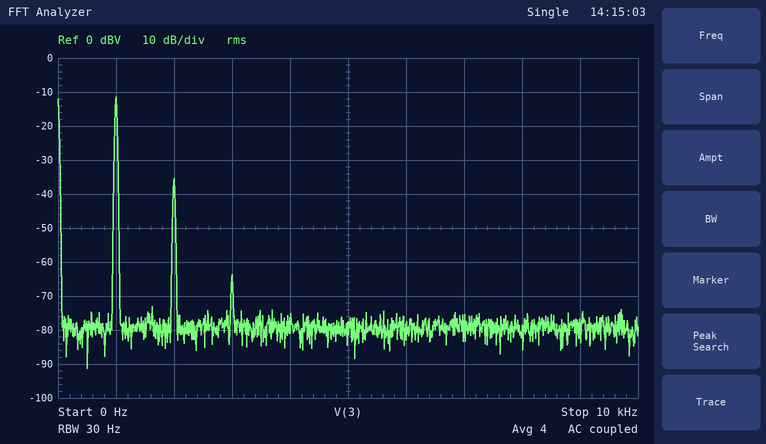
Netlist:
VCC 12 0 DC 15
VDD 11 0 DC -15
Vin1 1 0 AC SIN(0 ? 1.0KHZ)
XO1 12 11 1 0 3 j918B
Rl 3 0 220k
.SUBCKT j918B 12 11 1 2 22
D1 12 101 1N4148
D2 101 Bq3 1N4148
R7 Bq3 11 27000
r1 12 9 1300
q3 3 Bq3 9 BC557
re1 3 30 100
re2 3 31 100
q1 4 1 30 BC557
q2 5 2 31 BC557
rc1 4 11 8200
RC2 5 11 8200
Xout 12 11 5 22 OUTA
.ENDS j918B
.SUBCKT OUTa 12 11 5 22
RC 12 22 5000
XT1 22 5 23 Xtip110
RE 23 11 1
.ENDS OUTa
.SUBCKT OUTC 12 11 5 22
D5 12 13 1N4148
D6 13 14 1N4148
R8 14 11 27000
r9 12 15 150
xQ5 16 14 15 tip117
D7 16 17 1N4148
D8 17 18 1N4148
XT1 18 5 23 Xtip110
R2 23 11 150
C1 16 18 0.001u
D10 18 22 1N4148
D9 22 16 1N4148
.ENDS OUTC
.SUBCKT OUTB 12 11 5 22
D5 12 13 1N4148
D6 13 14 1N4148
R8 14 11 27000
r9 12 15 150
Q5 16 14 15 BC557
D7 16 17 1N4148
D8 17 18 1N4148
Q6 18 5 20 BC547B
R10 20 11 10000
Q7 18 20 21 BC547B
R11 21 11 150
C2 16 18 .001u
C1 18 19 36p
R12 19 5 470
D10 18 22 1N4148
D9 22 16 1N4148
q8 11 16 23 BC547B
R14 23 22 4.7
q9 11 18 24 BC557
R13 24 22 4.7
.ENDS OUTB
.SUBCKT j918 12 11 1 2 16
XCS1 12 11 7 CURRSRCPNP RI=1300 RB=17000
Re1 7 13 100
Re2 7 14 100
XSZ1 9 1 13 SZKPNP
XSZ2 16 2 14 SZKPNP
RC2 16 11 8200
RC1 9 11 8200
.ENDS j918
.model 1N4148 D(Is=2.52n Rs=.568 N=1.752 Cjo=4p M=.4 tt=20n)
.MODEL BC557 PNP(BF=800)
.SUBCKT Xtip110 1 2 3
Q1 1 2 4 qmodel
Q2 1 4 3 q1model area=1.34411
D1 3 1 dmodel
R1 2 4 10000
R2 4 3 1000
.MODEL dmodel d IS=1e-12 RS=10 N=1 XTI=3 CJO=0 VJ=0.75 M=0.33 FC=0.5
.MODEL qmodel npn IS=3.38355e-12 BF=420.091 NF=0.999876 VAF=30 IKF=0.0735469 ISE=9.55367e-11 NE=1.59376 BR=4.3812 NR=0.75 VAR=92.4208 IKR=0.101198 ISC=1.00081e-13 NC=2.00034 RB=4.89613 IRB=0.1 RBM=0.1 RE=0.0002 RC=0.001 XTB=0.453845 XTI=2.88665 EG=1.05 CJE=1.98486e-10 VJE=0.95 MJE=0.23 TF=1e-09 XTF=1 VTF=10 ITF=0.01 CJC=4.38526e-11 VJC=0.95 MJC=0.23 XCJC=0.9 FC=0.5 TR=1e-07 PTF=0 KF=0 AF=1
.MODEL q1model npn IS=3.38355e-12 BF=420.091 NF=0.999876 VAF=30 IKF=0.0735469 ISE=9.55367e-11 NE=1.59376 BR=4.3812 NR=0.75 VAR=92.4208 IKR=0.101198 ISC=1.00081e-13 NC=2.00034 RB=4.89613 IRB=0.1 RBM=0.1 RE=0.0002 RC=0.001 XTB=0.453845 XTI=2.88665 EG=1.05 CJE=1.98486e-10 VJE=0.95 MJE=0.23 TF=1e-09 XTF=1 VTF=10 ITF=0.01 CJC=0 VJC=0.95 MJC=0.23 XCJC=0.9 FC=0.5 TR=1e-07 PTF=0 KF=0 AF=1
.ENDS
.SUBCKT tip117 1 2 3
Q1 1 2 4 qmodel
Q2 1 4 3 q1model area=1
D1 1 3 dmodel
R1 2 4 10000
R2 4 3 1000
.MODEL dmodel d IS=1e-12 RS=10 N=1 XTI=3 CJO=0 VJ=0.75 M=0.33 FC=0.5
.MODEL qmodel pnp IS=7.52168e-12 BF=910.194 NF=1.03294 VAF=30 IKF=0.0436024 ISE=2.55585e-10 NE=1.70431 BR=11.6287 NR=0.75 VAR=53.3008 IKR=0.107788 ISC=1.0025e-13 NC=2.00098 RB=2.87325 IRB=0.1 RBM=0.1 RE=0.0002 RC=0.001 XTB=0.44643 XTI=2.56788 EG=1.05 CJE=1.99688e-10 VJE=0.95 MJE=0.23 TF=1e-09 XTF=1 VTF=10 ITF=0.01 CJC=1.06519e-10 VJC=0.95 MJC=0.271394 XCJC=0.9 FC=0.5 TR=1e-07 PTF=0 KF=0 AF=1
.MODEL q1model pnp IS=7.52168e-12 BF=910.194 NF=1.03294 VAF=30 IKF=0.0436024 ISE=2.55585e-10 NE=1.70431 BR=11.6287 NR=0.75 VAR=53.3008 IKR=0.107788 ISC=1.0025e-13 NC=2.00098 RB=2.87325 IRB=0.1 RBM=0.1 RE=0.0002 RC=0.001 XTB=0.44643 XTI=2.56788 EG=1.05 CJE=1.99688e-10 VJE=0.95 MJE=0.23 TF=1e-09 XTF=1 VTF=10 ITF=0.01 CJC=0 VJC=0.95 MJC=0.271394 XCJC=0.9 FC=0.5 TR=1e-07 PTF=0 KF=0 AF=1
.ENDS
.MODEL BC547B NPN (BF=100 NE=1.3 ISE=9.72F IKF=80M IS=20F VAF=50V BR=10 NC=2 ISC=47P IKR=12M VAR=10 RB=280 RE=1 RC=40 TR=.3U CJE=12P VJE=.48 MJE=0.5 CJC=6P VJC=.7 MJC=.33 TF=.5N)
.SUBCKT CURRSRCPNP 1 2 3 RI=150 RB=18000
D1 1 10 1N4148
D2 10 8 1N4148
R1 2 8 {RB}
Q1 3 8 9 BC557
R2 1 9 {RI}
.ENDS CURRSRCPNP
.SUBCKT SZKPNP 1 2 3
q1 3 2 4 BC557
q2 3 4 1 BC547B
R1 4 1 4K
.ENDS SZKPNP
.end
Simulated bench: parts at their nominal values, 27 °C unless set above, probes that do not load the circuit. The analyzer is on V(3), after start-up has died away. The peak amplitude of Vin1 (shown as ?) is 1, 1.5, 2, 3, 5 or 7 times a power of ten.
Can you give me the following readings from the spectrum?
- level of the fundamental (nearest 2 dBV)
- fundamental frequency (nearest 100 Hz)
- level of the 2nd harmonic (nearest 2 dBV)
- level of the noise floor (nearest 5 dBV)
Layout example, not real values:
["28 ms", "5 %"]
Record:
["-12 dBV", "1.0 kHz", "-36 dBV", "-80 dBV"]
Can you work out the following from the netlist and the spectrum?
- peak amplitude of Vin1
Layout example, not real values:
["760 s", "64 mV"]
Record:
["700 µV"]
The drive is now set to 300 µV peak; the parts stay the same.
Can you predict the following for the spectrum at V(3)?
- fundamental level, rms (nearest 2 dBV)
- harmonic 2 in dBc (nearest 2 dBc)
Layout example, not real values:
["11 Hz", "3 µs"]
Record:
["-18 dBV", "-32 dBc"]
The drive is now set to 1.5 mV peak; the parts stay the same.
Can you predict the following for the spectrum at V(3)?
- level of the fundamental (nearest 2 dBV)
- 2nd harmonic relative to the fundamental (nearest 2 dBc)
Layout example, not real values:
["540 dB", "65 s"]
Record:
["-4 dBV", "-18 dBc"]
